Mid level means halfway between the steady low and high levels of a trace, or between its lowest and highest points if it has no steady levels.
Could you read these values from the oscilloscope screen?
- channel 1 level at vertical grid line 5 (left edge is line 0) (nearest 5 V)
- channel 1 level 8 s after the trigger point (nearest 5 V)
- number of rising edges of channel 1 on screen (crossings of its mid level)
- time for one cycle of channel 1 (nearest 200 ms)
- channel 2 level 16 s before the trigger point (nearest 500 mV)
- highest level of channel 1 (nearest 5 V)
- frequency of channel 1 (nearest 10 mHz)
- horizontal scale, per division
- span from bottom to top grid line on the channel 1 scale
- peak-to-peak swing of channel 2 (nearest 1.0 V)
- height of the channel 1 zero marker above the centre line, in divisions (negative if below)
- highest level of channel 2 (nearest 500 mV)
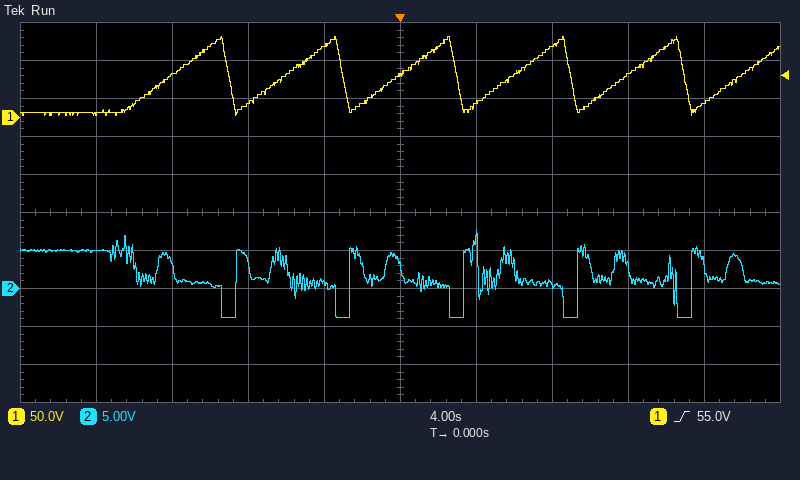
60 V
95 V
6
6.0 s
5.0 V
105 V
170 mHz
4 s
500 V
11.0 V
+2.5 div
7.5 V
